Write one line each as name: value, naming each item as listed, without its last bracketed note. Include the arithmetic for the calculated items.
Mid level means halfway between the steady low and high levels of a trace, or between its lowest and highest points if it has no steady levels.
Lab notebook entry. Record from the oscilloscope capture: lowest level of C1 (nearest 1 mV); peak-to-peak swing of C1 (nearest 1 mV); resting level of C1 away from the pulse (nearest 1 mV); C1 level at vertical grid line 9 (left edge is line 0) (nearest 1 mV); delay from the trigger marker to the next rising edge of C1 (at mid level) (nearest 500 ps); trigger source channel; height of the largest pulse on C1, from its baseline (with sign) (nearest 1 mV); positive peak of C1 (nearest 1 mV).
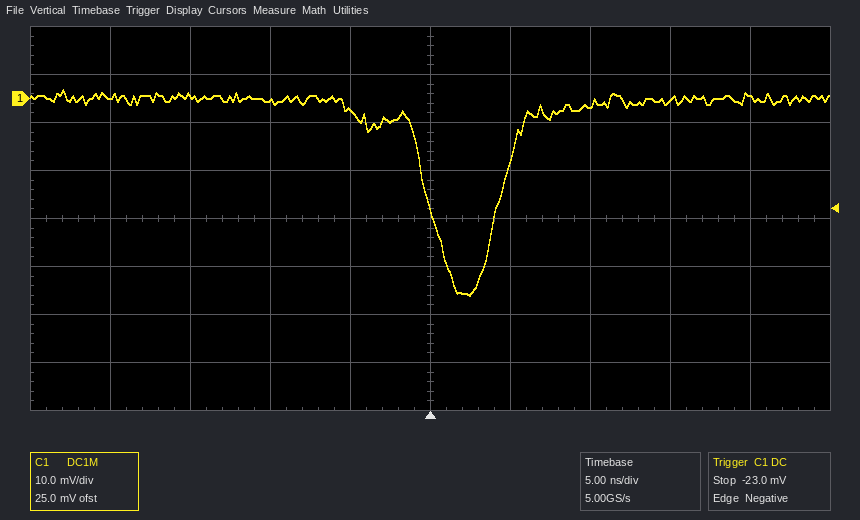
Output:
lowest level of C1: -41 mV
peak-to-peak swing of C1: 2 mV − (-41 mV) = 43 mV
resting level of C1 away from the pulse: 0 mV
C1 level at vertical grid line 9 (left edge is line 0): 0 mV
delay from the trigger marker to the next rising edge of C1 (at mid level): 4.5 ns
trigger source channel: C1
height of the largest pulse on C1, from its baseline (with sign): -41 mV − (0 mV) = -41 mV
positive peak of C1: 2 mV
